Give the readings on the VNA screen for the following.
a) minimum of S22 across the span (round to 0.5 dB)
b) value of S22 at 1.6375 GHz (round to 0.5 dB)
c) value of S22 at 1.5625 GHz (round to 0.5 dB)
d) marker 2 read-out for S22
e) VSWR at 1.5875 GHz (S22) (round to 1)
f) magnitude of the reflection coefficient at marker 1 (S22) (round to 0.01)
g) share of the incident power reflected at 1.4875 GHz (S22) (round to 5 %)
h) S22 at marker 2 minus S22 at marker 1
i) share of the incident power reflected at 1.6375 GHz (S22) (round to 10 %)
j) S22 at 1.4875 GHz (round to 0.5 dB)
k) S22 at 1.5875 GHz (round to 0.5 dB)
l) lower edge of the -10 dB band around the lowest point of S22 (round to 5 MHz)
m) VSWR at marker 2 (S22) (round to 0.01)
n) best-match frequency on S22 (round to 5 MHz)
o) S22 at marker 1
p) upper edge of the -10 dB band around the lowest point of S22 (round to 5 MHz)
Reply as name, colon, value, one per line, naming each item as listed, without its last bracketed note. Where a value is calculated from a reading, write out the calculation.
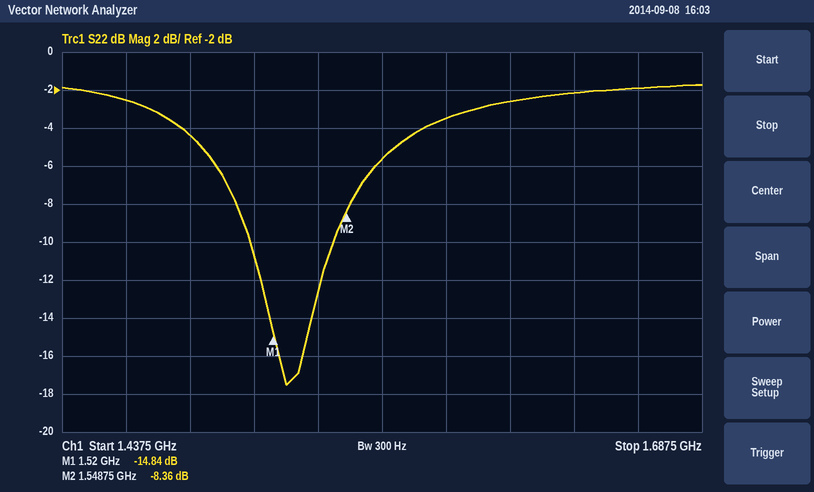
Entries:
minimum of S22 across the span: -17.5 dB
value of S22 at 1.6375 GHz: -2.0 dB
value of S22 at 1.5625 GHz: -5.5 dB
marker 2 read-out for S22: -8.36 dB
VSWR at 1.5875 GHz (S22): |Γ| = 10^(-3.5/20) = 0.6683; VSWR = (1 + 0.6683)/(1 − 0.6683) ≈ 5
magnitude of the reflection coefficient at marker 1 (S22): 10^(-14.84/20) ≈ 0.18
share of the incident power reflected at 1.4875 GHz (S22): 10^(-4.5/10) ≈ 35 %
S22 at marker 2 minus S22 at marker 1: -8.36 − (-14.84) = 6.48 dB
share of the incident power reflected at 1.6375 GHz (S22): 10^(-2/10) ≈ 63.1 %, so 60 % to the nearest 10 %
S22 at 1.4875 GHz: -4.5 dB
S22 at 1.5875 GHz: -3.5 dB
lower edge of the -10 dB band around the lowest point of S22: 1.510 GHz
VSWR at marker 2 (S22): (1 + 0.3819)/(1 − 0.3819) ≈ 2.24
best-match frequency on S22: 1.525 GHz
S22 at marker 1: -14.84 dB
upper edge of the -10 dB band around the lowest point of S22: 1.545 GHz
